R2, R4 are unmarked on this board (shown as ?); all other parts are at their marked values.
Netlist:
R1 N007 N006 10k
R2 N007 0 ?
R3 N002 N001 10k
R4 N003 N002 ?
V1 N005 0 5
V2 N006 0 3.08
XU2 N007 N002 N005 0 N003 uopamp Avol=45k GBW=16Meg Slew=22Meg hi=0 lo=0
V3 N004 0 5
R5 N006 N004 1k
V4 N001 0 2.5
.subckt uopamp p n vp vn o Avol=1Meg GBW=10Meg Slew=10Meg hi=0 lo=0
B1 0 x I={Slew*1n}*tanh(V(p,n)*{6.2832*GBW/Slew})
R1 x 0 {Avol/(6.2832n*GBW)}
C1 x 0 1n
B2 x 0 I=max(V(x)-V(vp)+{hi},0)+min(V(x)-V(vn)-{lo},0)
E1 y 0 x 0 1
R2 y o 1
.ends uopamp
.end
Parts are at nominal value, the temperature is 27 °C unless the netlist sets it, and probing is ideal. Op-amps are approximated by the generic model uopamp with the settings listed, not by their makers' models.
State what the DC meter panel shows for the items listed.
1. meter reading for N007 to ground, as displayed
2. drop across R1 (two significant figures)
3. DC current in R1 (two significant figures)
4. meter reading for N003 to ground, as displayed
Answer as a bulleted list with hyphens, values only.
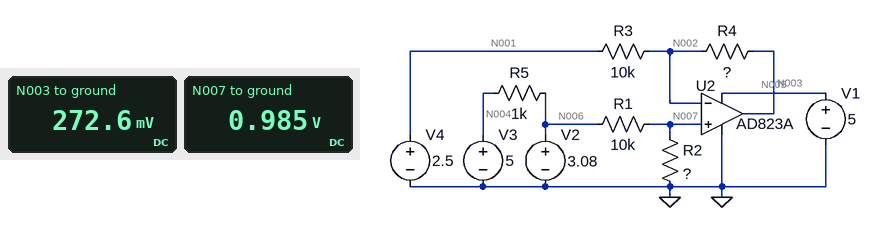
- 0.985 V
- 2.1 V
- 210 µA
- 272.6 mV
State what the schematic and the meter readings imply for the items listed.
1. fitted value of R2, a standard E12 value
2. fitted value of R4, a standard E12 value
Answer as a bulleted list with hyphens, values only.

- 4.7 kΩ
- 4.7 kΩ
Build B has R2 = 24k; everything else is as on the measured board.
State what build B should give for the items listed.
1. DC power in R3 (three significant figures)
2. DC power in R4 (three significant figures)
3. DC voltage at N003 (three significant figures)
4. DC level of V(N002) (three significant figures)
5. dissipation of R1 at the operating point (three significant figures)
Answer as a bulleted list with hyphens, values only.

- 10.6 µW
- 4.99 µW
- 2.02 V
- 2.17 V
- 82.1 µW
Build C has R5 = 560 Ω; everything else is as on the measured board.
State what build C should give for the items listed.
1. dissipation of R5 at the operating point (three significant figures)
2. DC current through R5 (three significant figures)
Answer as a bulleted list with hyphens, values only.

- 6.58 mW
- 3.43 mA
